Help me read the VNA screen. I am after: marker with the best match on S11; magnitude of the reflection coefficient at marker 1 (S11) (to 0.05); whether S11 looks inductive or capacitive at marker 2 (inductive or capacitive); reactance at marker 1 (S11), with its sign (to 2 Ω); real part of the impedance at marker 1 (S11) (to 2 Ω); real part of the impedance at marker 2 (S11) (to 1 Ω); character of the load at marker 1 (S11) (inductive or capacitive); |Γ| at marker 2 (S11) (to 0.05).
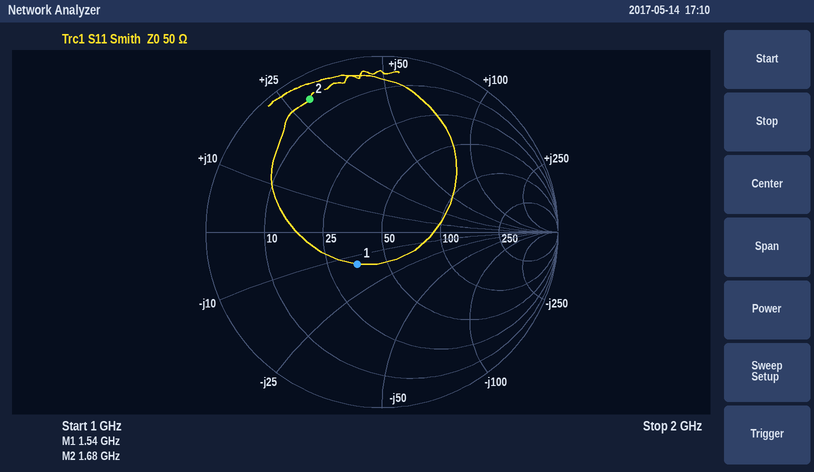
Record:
marker 1
0.25
inductive
-14 Ω
36 Ω
5 Ω
capacitive
0.85
